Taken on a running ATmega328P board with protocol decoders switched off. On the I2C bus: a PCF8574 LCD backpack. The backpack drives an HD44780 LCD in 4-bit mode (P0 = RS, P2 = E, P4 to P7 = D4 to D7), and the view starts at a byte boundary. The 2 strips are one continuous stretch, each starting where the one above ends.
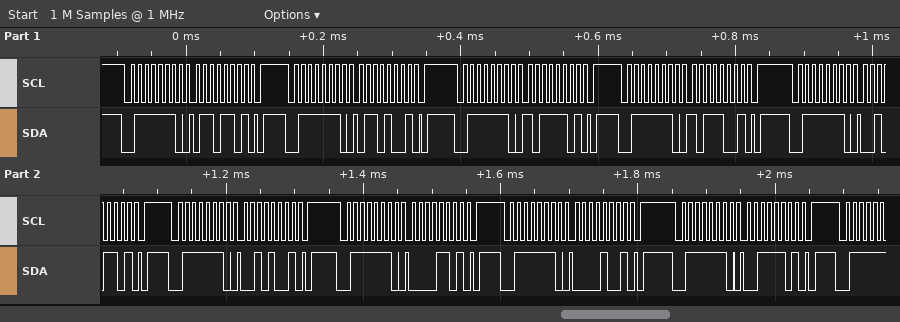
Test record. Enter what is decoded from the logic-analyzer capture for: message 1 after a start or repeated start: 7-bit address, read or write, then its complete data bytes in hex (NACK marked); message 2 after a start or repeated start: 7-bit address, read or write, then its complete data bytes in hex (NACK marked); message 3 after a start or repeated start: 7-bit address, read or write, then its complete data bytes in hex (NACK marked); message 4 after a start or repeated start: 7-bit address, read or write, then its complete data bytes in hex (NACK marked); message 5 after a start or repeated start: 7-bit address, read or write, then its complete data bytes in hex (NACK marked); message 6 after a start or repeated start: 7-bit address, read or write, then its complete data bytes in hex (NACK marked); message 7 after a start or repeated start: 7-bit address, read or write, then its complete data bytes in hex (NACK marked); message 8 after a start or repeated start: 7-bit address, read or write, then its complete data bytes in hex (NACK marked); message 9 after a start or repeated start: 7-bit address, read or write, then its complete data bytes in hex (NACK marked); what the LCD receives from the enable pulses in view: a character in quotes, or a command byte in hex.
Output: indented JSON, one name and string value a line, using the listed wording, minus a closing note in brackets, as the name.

{
  "message 1 after a start or repeated start: 7-bit address, read or write, then its complete data bytes in hex": "0x3F write: 6D",
  "message 2 after a start or repeated start: 7-bit address, read or write, then its complete data bytes in hex": "0x3F write: 69",
  "message 3 after a start or repeated start: 7-bit address, read or write, then its complete data bytes in hex": "0x3F write: BD",
  "message 4 after a start or repeated start: 7-bit address, read or write, then its complete data bytes in hex": "0x3F write: B9",
  "message 5 after a start or repeated start: 7-bit address, read or write, then its complete data bytes in hex": "0x3F write: 2D",
  "message 6 after a start or repeated start: 7-bit address, read or write, then its complete data bytes in hex": "0x3F write: 29",
  "message 7 after a start or repeated start: 7-bit address, read or write, then its complete data bytes in hex": "0x3F write: 0D",
  "message 8 after a start or repeated start: 7-bit address, read or write, then its complete data bytes in hex": "0x3F write: 09",
  "message 9 after a start or repeated start: 7-bit address, read or write, then its complete data bytes in hex": "0x3F write: 3D",
  "what the LCD receives from the enable pulses in view: a character in quotes, or a command byte in hex": "'k' ' '"
}
